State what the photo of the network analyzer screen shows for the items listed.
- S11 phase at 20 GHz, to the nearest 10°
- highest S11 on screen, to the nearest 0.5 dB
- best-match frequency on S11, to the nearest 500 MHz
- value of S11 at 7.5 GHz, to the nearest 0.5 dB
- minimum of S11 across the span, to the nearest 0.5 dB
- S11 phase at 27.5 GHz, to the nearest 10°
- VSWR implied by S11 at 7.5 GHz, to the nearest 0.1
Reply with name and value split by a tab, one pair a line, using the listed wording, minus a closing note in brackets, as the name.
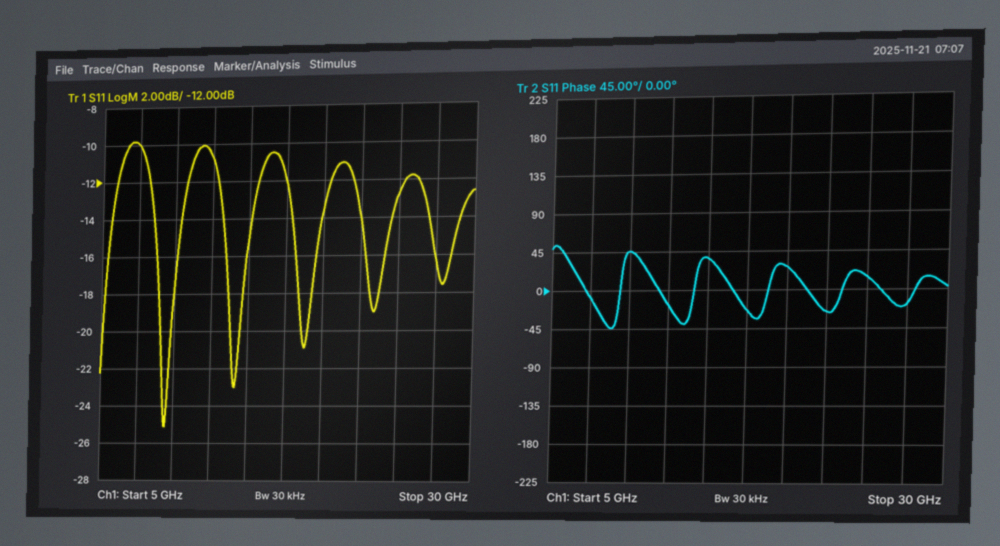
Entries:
S11 phase at 20 GHz, to the nearest 10°	30°
highest S11 on screen, to the nearest 0.5 dB	-10.0 dB
best-match frequency on S11, to the nearest 500 MHz	9.5 GHz
value of S11 at 7.5 GHz, to the nearest 0.5 dB	-10.0 dB
minimum of S11 across the span, to the nearest 0.5 dB	-25.0 dB
S11 phase at 27.5 GHz, to the nearest 10°	-20°
VSWR implied by S11 at 7.5 GHz, to the nearest 0.1	1.9
